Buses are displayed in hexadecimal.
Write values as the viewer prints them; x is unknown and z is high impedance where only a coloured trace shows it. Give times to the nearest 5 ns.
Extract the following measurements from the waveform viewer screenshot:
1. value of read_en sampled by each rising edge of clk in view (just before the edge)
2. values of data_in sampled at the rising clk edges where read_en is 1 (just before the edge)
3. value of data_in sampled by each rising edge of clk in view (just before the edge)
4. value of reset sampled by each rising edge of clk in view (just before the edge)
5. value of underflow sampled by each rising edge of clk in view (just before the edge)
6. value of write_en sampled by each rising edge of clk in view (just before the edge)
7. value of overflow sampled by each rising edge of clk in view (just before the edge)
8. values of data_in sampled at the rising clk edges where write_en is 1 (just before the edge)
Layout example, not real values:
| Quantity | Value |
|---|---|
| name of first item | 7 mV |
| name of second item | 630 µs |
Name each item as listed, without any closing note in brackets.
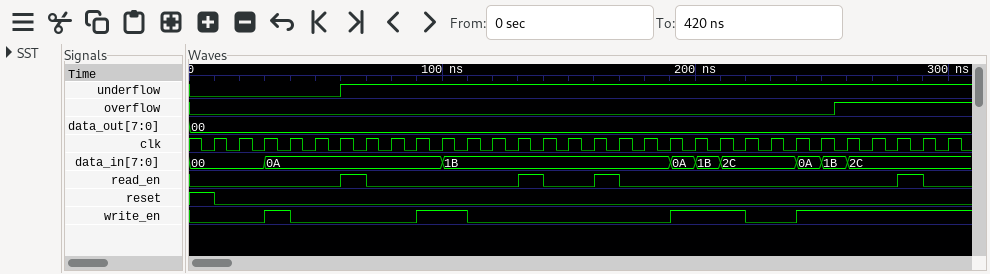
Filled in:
| Quantity | Value |
|---|---|
| value of read_en sampled by each rising edge of clk in view | 0 0 0 0 0 0 1 0 0 0 0 0 0 1 0 0 1 0 0 0 0 0 0 0 0 0 0 0 1 0 |
| values of data_in sampled at the rising clk edges where read_en is 1 | 0A, 1B, 1B, 2C |
| value of data_in sampled by each rising edge of clk in view | 00, 00, 00, 0A, 0A, 0A, 0A, 0A, 0A, 0A, 1B, 1B, 1B, 1B, 1B, 1B, 1B, 1B, 1B, 0A, 1B, 2C, 2C, 2C, 0A, 1B, 2C, 2C, 2C, 2C |
| value of reset sampled by each rising edge of clk in view | 1 0 0 0 0 0 0 0 0 0 0 0 0 0 0 0 0 0 0 0 0 0 0 0 0 0 0 0 0 0 |
| value of underflow sampled by each rising edge of clk in view | 0 0 0 0 0 0 1 1 1 1 1 1 1 1 1 1 1 1 1 1 1 1 1 1 1 1 1 1 1 1 |
| value of write_en sampled by each rising edge of clk in view | 0 0 0 1 0 0 0 0 0 1 1 0 0 0 0 0 0 0 0 1 1 1 0 0 1 1 1 1 1 1 |
| value of overflow sampled by each rising edge of clk in view | 0 0 0 0 0 0 0 0 0 0 0 0 0 0 0 0 0 0 0 0 0 0 0 0 0 1 1 1 1 1 |
| values of data_in sampled at the rising clk edges where write_en is 1 | 0A, 0A, 1B, 0A, 1B, 2C, 0A, 1B, 2C, 2C, 2C, 2C |
